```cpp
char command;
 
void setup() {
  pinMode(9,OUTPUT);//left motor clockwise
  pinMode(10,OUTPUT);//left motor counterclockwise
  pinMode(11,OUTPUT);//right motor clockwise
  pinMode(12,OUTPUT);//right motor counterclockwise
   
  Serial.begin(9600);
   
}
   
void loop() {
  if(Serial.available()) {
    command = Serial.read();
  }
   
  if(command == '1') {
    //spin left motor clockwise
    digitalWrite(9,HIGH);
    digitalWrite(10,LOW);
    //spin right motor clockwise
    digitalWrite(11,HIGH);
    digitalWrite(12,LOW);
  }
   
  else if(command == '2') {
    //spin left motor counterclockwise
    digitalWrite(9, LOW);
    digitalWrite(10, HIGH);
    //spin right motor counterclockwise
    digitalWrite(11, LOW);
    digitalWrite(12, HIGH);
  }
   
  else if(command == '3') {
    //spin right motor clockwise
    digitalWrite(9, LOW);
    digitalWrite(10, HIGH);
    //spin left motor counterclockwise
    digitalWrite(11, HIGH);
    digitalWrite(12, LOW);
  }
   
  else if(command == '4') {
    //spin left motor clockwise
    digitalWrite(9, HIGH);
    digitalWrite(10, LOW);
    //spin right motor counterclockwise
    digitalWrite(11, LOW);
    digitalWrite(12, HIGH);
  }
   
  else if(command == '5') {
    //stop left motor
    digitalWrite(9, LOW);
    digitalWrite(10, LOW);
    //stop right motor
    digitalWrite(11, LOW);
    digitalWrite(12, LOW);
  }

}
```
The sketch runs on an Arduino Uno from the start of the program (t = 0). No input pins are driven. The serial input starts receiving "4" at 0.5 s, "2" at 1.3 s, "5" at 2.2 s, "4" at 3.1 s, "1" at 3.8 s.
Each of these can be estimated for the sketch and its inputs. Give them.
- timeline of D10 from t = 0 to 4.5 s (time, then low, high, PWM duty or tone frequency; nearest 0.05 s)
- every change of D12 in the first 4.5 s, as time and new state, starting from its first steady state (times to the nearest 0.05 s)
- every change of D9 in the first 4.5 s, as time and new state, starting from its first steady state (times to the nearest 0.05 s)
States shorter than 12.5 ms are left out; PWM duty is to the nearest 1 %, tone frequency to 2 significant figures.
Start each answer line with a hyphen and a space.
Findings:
- 0 s low; 1.3 s high; 2.2 s low
- 0 s low; 0.5 s high; 2.2 s low; 3.1 s high; 3.8 s low
- 0 s low; 0.5 s high; 1.3 s low; 3.1 s high
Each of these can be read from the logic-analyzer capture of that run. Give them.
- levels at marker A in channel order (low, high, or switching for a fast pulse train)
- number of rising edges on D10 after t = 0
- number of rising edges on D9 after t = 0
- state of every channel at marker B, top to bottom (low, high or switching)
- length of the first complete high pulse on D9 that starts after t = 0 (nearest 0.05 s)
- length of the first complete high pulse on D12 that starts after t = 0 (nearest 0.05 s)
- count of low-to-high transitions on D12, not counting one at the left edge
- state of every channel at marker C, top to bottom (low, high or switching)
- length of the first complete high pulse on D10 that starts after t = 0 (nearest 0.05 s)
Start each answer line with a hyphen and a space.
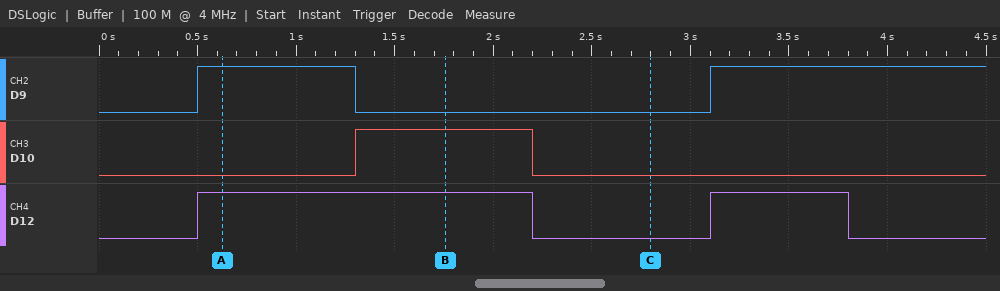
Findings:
- D9 high, D10 low, D12 high
- 1
- 2
- D9 low, D10 high, D12 high
- 0.80 s
- 1.70 s
- 2
- D9 low, D10 low, D12 low
- 0.90 s
